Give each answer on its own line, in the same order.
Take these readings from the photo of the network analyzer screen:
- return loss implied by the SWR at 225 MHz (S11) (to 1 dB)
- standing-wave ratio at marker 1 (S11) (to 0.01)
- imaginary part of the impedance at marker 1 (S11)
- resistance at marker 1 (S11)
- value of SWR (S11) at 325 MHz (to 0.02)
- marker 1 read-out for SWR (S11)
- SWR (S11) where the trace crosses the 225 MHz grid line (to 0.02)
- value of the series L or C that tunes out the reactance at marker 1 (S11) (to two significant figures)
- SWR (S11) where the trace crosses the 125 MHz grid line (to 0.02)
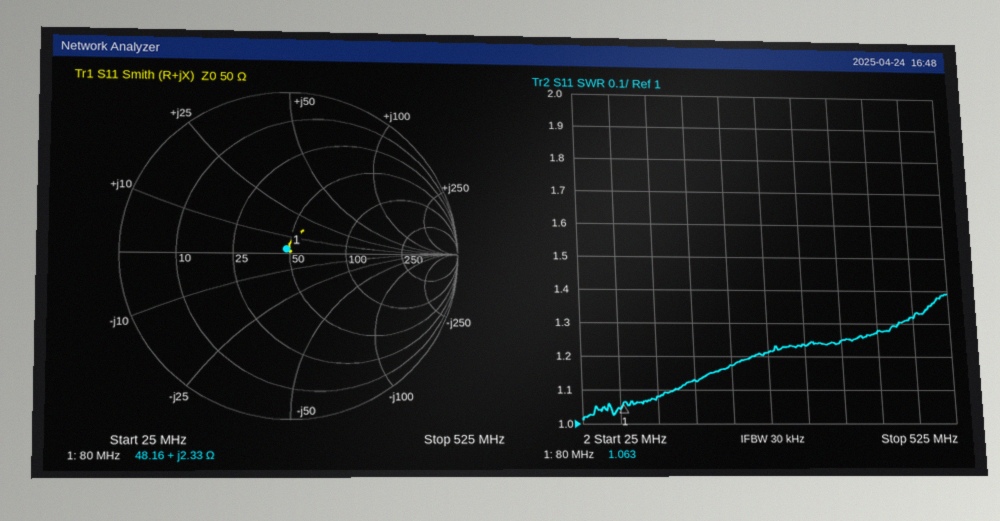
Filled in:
22 dB
1.06
+2.33 Ω
48.16 Ω
1.24
1.063
1.18
850 pF
1.08
